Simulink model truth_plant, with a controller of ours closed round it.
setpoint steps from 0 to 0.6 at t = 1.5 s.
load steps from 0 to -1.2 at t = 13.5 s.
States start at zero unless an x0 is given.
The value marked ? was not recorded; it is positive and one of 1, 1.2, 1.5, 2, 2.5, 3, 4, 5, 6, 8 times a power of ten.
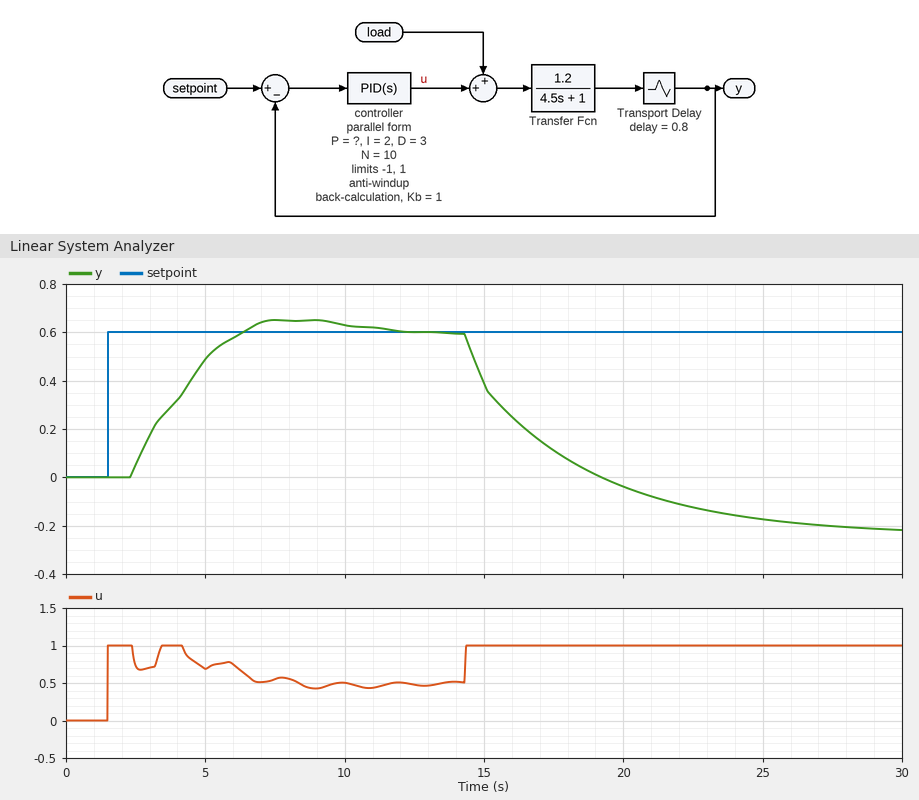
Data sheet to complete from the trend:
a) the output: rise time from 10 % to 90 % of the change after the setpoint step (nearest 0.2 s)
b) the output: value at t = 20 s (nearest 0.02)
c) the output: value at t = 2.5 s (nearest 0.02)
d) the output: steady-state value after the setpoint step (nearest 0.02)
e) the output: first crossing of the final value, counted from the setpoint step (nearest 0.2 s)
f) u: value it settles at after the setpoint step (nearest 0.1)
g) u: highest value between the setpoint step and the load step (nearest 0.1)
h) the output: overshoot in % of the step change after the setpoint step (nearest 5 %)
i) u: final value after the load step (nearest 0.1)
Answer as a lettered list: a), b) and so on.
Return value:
a) 3.0 s
b) -0.04
c) 0.06
d) 0.60
e) 4.8 s
f) 0.5
g) 1.0
h) 10 %
i) 1.0
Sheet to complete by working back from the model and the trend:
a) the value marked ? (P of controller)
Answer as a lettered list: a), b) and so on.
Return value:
a) 4
